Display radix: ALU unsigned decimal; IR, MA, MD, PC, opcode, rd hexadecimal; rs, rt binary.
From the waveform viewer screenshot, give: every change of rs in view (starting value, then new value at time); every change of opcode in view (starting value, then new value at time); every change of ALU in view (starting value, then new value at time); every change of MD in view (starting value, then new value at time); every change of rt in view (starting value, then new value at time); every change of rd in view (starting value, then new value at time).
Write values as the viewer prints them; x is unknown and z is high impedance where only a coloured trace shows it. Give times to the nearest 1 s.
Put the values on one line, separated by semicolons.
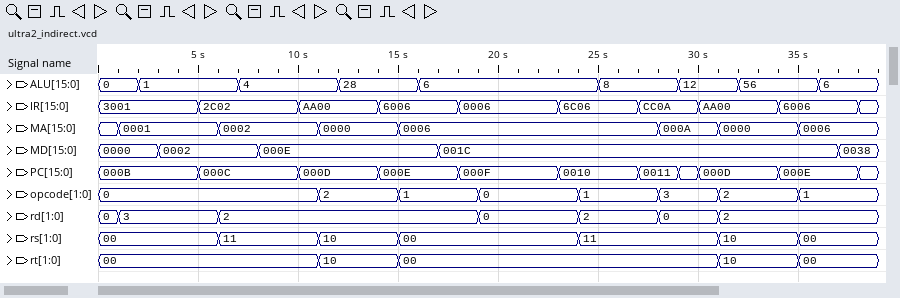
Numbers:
00, 11 at 6 s, 10 at 11 s, 00 at 15 s, 11 at 24 s, 10 at 31 s, 00 at 35 s; 0, 2 at 11 s, 1 at 15 s, 0 at 19 s, 1 at 24 s, 3 at 28 s, 2 at 31 s, 1 at 35 s; 0, 1 at 2 s, 4 at 7 s, 28 at 12 s, 6 at 16 s, 8 at 25 s, 12 at 29 s, 56 at 32 s, 6 at 36 s; 0000, 0002 at 3 s, 000E at 8 s, 001C at 17 s, 0038 at 37 s; 00, 10 at 11 s, 00 at 15 s, 10 at 31 s, 00 at 35 s; 0, 3 at 1 s, 2 at 6 s, 0 at 19 s, 2 at 24 s, 0 at 28 s, 2 at 31 s
